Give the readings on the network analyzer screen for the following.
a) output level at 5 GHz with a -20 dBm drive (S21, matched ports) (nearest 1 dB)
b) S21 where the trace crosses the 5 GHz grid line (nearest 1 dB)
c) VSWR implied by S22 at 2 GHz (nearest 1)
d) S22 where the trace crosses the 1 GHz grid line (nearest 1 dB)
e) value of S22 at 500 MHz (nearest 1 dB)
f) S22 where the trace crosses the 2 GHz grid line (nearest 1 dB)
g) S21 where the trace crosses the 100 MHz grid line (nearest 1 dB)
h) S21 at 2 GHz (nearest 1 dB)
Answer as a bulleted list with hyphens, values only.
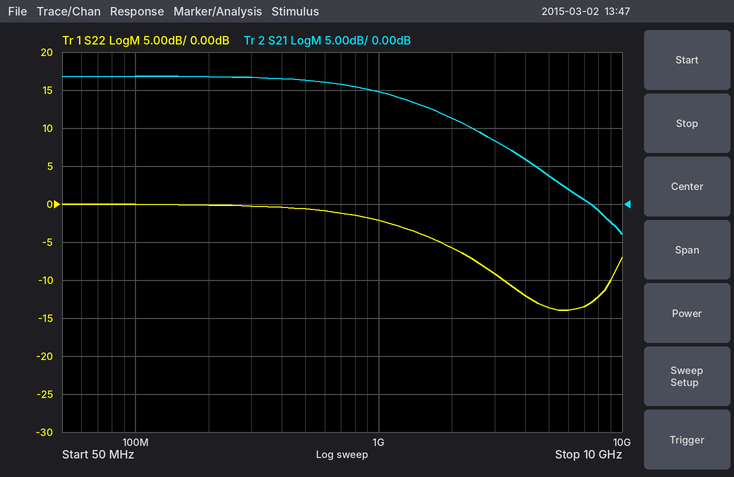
- -16 dBm
- 4 dB
- 3
- -2 dB
- -1 dB
- -6 dB
- 17 dB
- 11 dB
